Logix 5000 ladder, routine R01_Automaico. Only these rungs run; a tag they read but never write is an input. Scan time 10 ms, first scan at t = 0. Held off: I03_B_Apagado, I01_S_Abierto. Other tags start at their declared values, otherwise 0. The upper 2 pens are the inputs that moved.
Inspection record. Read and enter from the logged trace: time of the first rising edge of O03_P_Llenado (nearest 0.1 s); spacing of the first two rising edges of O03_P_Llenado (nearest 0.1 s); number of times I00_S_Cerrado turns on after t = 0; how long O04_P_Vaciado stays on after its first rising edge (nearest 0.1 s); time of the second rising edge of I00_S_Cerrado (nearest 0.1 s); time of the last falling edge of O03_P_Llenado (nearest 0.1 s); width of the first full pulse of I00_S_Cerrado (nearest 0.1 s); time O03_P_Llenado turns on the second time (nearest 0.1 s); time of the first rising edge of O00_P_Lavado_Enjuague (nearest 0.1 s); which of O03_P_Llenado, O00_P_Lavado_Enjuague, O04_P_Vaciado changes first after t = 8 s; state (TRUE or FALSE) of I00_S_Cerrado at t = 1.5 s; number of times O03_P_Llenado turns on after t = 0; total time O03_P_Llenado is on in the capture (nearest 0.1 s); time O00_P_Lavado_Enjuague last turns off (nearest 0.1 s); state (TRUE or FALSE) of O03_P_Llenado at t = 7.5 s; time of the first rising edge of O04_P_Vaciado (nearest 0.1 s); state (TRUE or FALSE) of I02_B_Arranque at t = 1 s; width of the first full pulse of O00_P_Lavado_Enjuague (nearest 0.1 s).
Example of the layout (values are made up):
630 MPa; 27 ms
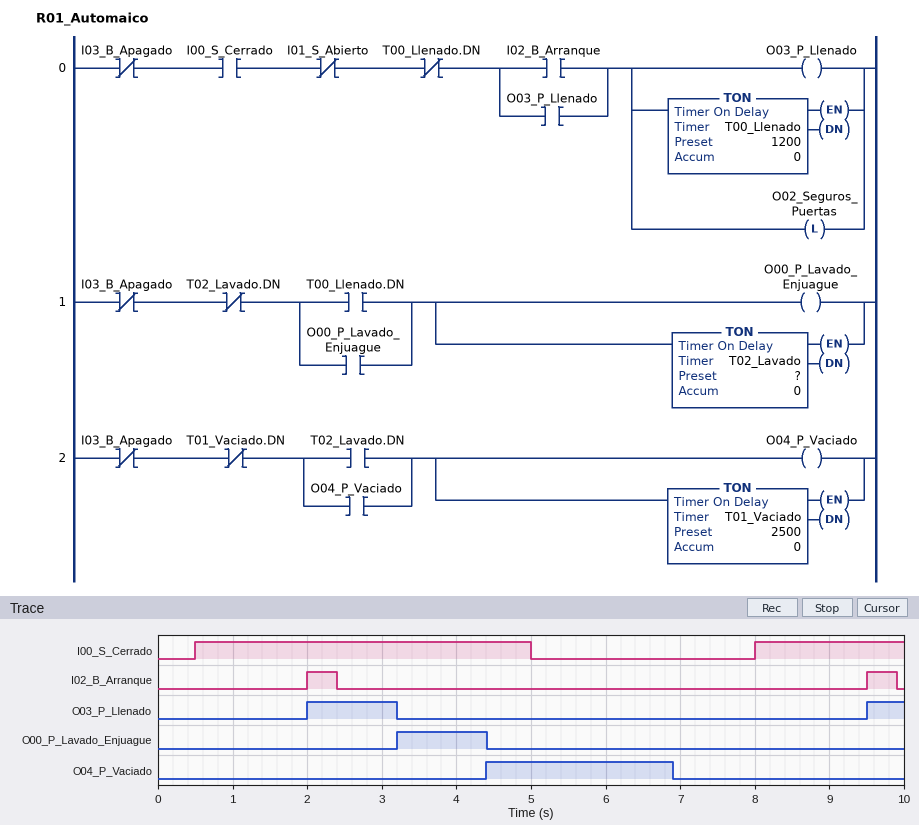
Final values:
2.0 s; 7.5 s; 2; 2.5 s; 8.0 s; 3.2 s; 4.5 s; 9.5 s; 3.2 s; O03_P_Llenado; TRUE; 2; 1.7 s; 4.4 s; FALSE; 4.4 s; FALSE; 1.2 s
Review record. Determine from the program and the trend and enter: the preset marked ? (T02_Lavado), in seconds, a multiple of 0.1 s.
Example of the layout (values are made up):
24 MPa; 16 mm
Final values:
1.2 s
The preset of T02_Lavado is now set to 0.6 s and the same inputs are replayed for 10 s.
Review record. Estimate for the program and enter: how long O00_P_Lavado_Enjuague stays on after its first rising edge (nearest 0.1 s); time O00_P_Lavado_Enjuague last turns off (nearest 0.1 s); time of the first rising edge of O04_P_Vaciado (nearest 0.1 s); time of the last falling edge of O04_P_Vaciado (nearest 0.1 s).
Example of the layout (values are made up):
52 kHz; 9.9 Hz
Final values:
0.6 s; 3.8 s; 3.8 s; 6.3 s
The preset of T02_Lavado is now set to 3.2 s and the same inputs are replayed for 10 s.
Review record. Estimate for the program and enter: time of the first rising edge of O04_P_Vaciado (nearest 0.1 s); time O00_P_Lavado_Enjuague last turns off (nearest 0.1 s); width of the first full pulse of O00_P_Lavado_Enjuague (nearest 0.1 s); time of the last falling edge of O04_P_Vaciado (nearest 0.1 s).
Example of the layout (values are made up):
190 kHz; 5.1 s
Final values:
6.4 s; 6.4 s; 3.2 s; 8.9 s
